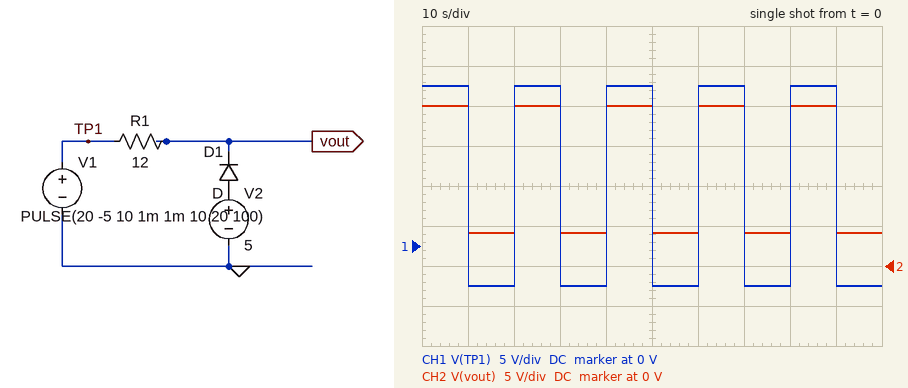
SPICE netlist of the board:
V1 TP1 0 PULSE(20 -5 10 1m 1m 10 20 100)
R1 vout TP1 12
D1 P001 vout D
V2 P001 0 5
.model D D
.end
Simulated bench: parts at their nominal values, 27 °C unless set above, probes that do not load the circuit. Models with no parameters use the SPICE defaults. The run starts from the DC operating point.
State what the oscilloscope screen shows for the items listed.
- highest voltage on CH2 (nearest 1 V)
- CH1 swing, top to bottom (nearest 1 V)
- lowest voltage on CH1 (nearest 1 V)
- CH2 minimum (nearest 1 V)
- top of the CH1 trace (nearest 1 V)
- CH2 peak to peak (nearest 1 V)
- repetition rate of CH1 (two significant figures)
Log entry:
20 V
25 V
-5 V
4 V
20 V
16 V
50 mHz
